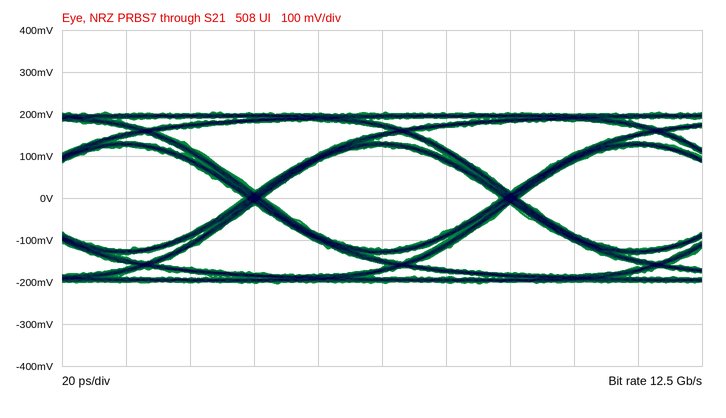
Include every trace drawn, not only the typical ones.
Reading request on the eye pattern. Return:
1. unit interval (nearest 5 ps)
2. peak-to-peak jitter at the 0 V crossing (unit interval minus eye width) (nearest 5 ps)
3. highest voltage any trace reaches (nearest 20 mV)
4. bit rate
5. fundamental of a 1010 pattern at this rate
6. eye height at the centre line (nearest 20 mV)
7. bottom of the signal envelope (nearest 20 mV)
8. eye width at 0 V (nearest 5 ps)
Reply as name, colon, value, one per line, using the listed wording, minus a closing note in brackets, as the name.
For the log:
unit interval: 80 ps
peak-to-peak jitter at the 0 V crossing (unit interval minus eye width): 5 ps
highest voltage any trace reaches: 200 mV
bit rate: 12.5 Gb/s
fundamental of a 1010 pattern at this rate: 6.25 GHz
eye height at the centre line: 240 mV
bottom of the signal envelope: -200 mV
eye width at 0 V: 75 ps
